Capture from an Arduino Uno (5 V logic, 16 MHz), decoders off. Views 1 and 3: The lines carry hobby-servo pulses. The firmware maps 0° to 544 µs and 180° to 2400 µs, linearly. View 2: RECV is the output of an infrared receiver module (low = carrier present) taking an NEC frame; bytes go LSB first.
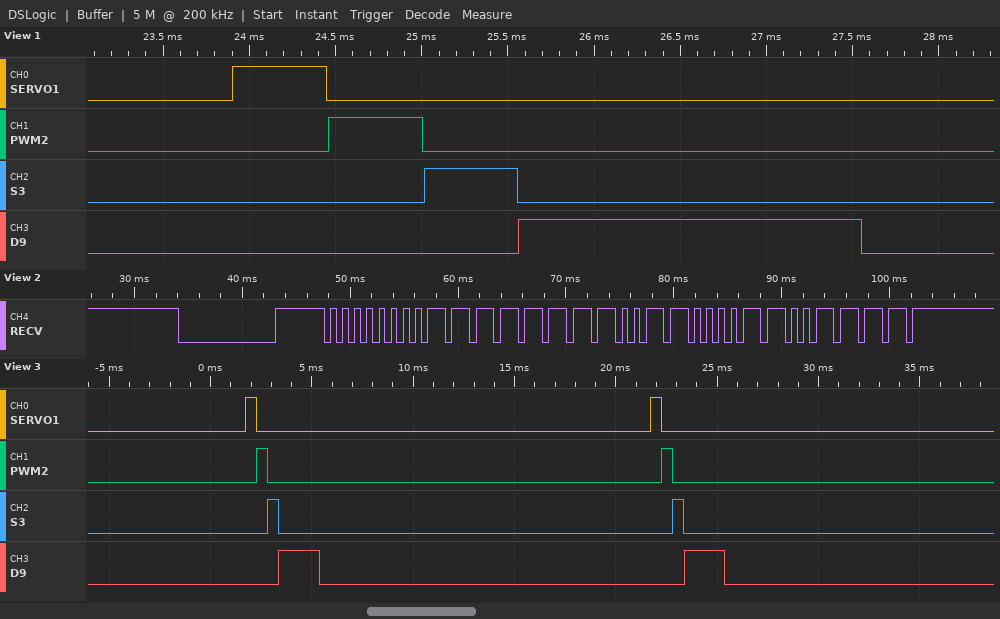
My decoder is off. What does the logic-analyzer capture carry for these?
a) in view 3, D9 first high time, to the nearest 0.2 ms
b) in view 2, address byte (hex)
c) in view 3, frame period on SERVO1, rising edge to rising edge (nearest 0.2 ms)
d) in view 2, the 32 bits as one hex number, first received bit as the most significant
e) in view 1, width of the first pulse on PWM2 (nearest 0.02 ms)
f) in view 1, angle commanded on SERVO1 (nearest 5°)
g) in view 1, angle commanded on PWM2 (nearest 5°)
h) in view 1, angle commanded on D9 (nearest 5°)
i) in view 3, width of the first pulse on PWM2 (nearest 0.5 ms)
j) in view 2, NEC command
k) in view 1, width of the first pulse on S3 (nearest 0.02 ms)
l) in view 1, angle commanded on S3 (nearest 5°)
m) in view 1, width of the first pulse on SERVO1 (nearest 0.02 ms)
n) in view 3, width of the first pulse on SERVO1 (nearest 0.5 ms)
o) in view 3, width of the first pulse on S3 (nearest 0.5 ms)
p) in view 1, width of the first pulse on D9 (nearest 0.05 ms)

2.0 ms
0x00
20.0 ms
0x00FF30CF
0.54 ms
0°
0°
140°
0.5 ms
0x0C
0.54 ms
0°
0.54 ms
0.5 ms
0.5 ms
2.00 ms
